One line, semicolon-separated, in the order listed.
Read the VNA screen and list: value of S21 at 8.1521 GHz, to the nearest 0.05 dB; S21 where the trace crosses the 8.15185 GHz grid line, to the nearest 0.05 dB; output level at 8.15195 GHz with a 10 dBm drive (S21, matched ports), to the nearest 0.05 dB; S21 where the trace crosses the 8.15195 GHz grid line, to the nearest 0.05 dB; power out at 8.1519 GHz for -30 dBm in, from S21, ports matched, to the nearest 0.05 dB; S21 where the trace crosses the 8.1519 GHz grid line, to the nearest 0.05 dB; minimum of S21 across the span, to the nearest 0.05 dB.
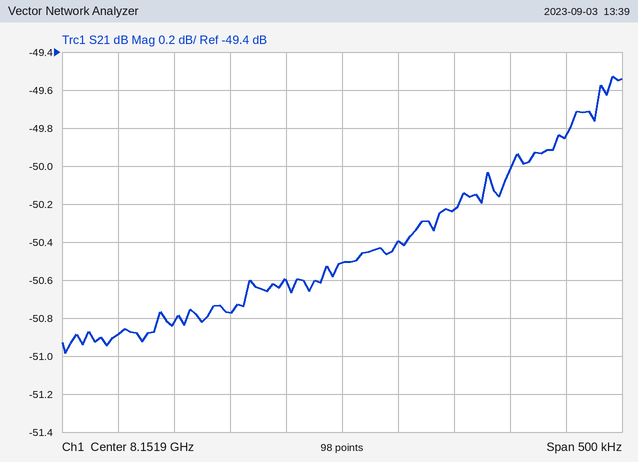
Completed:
-49.85 dB; -50.60 dB; -40.40 dBm; -50.40 dB; -80.50 dBm; -50.50 dB; -51.00 dB
